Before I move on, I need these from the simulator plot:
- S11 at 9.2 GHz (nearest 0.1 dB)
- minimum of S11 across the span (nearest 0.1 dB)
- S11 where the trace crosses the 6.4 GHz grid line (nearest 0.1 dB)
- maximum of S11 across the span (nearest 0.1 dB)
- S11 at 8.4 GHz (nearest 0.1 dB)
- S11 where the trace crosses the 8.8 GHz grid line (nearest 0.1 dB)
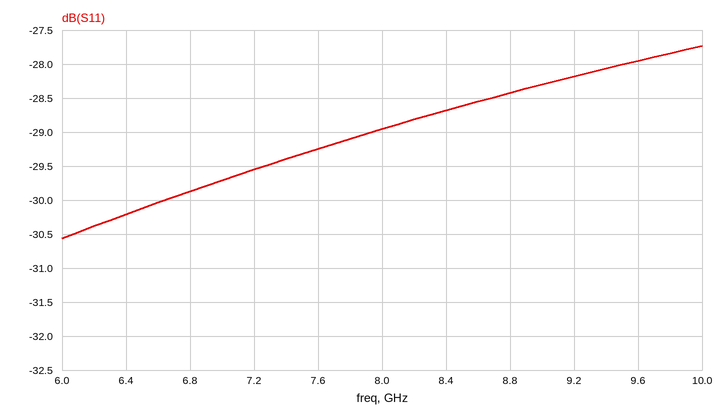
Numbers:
-28.2 dB
-30.6 dB
-30.2 dB
-27.7 dB
-28.7 dB
-28.4 dB
